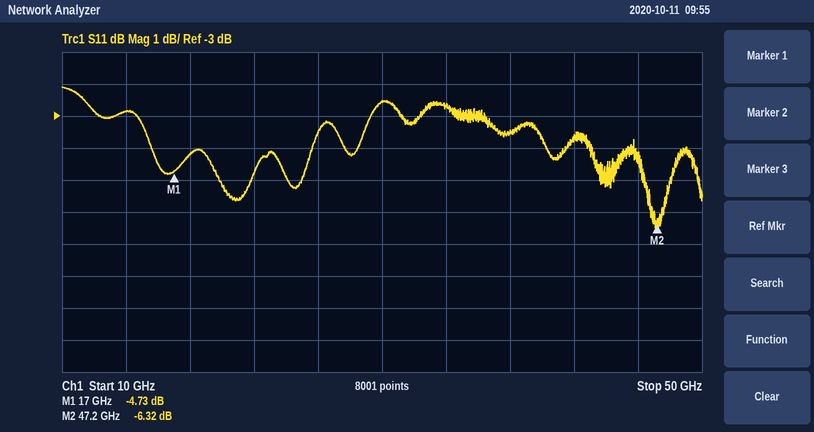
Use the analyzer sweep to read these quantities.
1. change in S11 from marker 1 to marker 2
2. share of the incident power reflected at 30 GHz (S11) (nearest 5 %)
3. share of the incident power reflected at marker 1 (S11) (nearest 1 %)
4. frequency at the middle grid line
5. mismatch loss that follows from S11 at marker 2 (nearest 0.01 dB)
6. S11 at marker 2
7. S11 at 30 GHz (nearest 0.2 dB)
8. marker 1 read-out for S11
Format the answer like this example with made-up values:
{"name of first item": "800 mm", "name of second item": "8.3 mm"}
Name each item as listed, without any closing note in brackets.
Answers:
{"change in S11 from marker 1 to marker 2": "-1.59 dB", "share of the incident power reflected at 30 GHz (S11)": "55 %", "share of the incident power reflected at marker 1 (S11)": "34 %", "frequency at the middle grid line": "30 GHz", "mismatch loss that follows from S11 at marker 2": "1.15 dB", "S11 at marker 2": "-6.32 dB", "S11 at 30 GHz": "-2.6 dB", "marker 1 read-out for S11": "-4.73 dB"}
